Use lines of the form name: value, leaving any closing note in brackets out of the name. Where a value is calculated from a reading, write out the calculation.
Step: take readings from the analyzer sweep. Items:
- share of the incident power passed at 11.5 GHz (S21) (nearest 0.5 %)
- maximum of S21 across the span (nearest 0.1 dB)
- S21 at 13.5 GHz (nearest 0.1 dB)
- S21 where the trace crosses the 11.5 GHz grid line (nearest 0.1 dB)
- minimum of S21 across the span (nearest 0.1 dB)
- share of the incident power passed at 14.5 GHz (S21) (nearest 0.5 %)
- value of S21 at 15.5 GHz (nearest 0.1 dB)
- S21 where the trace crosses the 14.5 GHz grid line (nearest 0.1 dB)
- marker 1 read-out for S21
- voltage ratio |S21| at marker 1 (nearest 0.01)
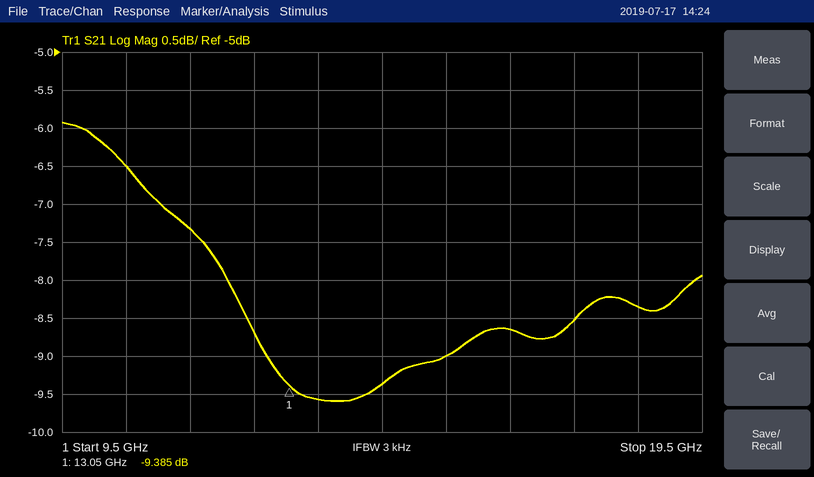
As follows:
share of the incident power passed at 11.5 GHz (S21): 10^(-7.3/10) ≈ 18.6 %, so 18.5 % to the nearest 0.5 %
maximum of S21 across the span: -5.9 dB
S21 at 13.5 GHz: -9.6 dB
S21 where the trace crosses the 11.5 GHz grid line: -7.3 dB
minimum of S21 across the span: -9.6 dB
share of the incident power passed at 14.5 GHz (S21): 10^(-9.4/10) ≈ 11.5 %
value of S21 at 15.5 GHz: -9.0 dB
S21 where the trace crosses the 14.5 GHz grid line: -9.4 dB
marker 1 read-out for S21: -9.385 dB
voltage ratio |S21| at marker 1: 10^(-9.385/20) ≈ 0.34
